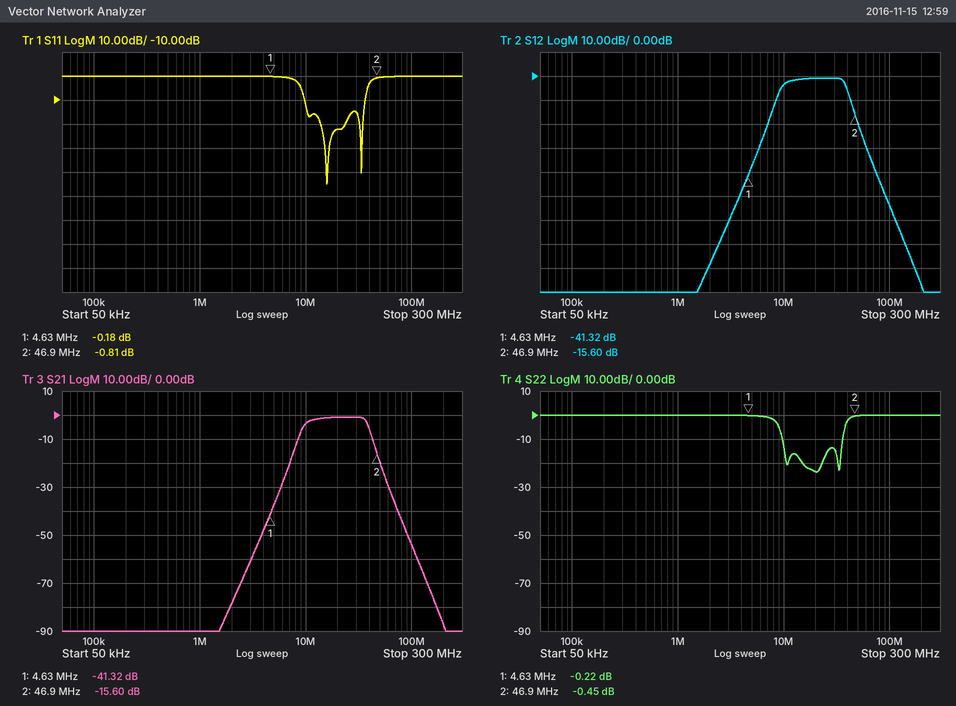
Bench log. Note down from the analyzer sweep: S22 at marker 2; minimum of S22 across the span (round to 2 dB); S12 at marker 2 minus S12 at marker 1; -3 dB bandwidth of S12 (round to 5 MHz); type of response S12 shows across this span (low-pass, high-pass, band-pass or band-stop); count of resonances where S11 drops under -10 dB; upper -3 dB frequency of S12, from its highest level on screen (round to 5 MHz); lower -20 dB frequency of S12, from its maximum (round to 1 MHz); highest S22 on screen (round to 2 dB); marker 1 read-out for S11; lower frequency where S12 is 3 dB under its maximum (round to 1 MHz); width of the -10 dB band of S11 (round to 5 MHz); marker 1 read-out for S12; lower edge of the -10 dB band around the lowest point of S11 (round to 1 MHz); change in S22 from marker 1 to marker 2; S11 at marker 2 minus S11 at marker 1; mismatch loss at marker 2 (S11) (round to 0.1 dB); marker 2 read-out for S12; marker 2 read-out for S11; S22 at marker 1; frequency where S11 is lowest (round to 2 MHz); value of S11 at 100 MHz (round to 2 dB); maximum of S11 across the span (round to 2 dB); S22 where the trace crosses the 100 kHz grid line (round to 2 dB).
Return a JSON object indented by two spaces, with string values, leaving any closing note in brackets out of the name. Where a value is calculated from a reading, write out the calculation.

{
  "S22 at marker 2": "-0.45 dB",
  "minimum of S22 across the span": "-24 dB",
  "S12 at marker 2 minus S12 at marker 1": "-15.6 − (-41.32) = 25.72 dB",
  "-3 dB bandwidth of S12": "40 MHz − 10 MHz = 30 MHz",
  "type of response S12 shows across this span": "band-pass",
  "count of resonances where S11 drops under -10 dB": "2",
  "upper -3 dB frequency of S12, from its highest level on screen": "40 MHz",
  "lower -20 dB frequency of S12, from its maximum": "7 MHz",
  "highest S22 on screen": "0 dB",
  "marker 1 read-out for S11": "-0.18 dB",
  "lower frequency where S12 is 3 dB under its maximum": "10 MHz",
  "width of the -10 dB band of S11": "35 MHz − 10 MHz = 25 MHz",
  "marker 1 read-out for S12": "-41.32 dB",
  "lower edge of the -10 dB band around the lowest point of S11": "10 MHz",
  "change in S22 from marker 1 to marker 2": "-0.45 − (-0.22) = -0.23 dB",
  "S11 at marker 2 minus S11 at marker 1": "-0.81 − (-0.18) = -0.63 dB",
  "mismatch loss at marker 2 (S11)": "−10 log10(1 − 10^(-0.81/10)) ≈ 7.7 dB",
  "marker 2 read-out for S12": "-15.60 dB",
  "marker 2 read-out for S11": "-0.81 dB",
  "S22 at marker 1": "-0.22 dB",
  "frequency where S11 is lowest": "16 MHz",
  "value of S11 at 100 MHz": "0 dB",
  "maximum of S11 across the span": "0 dB",
  "S22 where the trace crosses the 100 kHz grid line": "0 dB"
}
